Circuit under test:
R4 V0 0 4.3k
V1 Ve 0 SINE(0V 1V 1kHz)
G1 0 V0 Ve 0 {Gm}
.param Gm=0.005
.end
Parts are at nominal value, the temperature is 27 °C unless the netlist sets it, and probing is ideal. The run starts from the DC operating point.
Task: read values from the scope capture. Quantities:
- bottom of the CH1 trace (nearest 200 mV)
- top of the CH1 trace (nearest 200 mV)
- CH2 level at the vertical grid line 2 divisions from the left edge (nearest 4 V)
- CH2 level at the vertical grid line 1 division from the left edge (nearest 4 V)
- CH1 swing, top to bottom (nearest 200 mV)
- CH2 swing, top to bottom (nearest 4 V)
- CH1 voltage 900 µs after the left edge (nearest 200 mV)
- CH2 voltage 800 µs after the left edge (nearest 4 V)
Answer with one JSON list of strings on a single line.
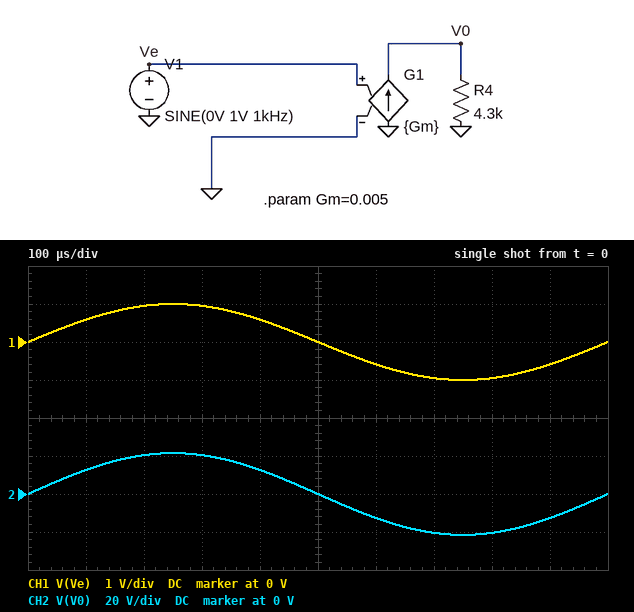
["-1.0 V", "1.0 V", "20 V", "12 V", "2.0 V", "44 V", "-600 mV", "-20 V"]
